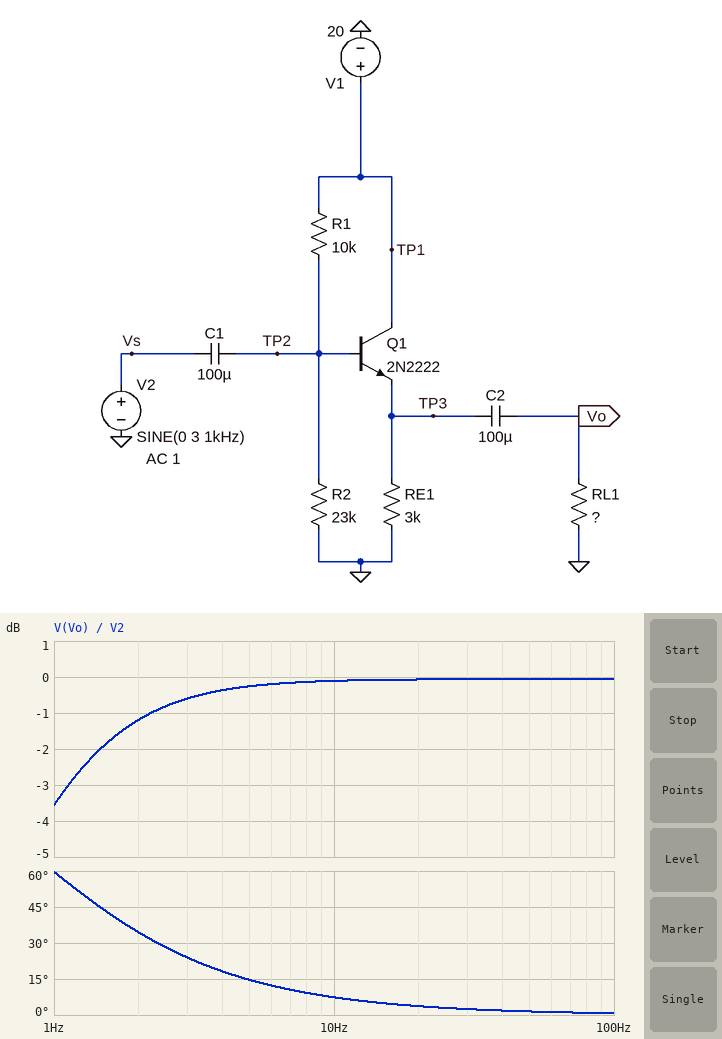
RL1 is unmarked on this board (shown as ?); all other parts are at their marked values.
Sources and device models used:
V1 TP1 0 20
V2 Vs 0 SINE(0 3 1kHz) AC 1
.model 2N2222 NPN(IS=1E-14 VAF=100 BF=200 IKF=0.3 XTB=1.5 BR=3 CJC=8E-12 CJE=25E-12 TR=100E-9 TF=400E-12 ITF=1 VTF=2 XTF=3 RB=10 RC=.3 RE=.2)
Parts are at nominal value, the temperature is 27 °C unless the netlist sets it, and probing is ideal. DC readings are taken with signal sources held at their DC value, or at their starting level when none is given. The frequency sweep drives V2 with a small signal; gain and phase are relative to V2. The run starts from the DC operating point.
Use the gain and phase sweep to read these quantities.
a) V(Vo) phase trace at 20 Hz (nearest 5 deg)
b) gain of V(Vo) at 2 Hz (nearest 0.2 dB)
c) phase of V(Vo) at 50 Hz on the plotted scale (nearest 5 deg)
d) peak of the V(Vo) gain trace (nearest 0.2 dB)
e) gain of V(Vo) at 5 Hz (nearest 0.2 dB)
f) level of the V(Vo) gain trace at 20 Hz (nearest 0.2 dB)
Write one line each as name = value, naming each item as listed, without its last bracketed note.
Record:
V(Vo) phase trace at 20 Hz = 5 deg
gain of V(Vo) at 2 Hz = -1.2 dB
phase of V(Vo) at 50 Hz on the plotted scale = 0 deg
peak of the V(Vo) gain trace = 0 dB
gain of V(Vo) at 5 Hz = -0.2 dB
level of the V(Vo) gain trace at 20 Hz = 0 dB
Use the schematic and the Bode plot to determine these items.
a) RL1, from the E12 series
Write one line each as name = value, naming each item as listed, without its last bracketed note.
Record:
RL1, from the E12 series = 1.5 kΩ
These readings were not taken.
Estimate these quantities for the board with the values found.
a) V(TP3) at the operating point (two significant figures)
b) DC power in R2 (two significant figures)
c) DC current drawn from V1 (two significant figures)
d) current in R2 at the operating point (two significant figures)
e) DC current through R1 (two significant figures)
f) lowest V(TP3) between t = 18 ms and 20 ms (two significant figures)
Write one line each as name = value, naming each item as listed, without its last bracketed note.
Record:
V(TP3) at the operating point = 13 V
DC power in R2 = 8.3 mW
DC current drawn from V1 = 5.0 mA
current in R2 at the operating point = 600 µA
DC current through R1 = 620 µA
lowest V(TP3) between t = 18 ms and 20 ms = 10 V
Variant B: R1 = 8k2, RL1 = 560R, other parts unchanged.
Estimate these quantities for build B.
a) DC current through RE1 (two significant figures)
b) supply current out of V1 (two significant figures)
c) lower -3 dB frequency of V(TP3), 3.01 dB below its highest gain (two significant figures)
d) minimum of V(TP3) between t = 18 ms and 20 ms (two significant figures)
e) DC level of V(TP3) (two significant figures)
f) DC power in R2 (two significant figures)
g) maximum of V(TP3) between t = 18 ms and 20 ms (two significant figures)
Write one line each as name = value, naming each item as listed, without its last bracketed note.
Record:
DC current through RE1 = 4.6 mA
supply current out of V1 = 5.3 mA
lower -3 dB frequency of V(TP3), 3.01 dB below its highest gain = 260 mHz
minimum of V(TP3) between t = 18 ms and 20 ms = 12 V
DC level of V(TP3) = 14 V
DC power in R2 = 9.3 mW
maximum of V(TP3) between t = 18 ms and 20 ms = 17 V
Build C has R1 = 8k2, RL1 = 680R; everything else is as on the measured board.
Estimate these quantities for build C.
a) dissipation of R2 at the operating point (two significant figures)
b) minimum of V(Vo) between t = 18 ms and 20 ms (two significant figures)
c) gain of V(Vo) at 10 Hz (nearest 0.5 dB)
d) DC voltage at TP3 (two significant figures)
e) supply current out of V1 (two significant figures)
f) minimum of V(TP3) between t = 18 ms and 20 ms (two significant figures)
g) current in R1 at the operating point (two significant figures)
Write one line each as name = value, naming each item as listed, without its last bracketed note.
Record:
dissipation of R2 at the operating point = 9.3 mW
minimum of V(Vo) between t = 18 ms and 20 ms = -2.6 V
gain of V(Vo) at 10 Hz = -0.5 dB
DC voltage at TP3 = 14 V
supply current out of V1 = 5.3 mA
minimum of V(TP3) between t = 18 ms and 20 ms = 11 V
current in R1 at the operating point = 660 µA
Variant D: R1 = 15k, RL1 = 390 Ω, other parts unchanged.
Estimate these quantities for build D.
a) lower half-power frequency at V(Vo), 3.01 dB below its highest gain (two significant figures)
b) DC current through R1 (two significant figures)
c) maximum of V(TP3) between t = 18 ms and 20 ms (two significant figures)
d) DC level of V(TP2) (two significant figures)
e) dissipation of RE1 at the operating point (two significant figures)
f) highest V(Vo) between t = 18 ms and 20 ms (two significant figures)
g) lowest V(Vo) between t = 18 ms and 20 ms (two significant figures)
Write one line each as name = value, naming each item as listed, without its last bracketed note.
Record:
lower half-power frequency at V(Vo), 3.01 dB below its highest gain = 4.0 Hz
DC current through R1 = 540 µA
maximum of V(TP3) between t = 18 ms and 20 ms = 14 V
DC level of V(TP2) = 12 V
dissipation of RE1 at the operating point = 42 mW
highest V(Vo) between t = 18 ms and 20 ms = 2.8 V
lowest V(Vo) between t = 18 ms and 20 ms = -1.3 V
